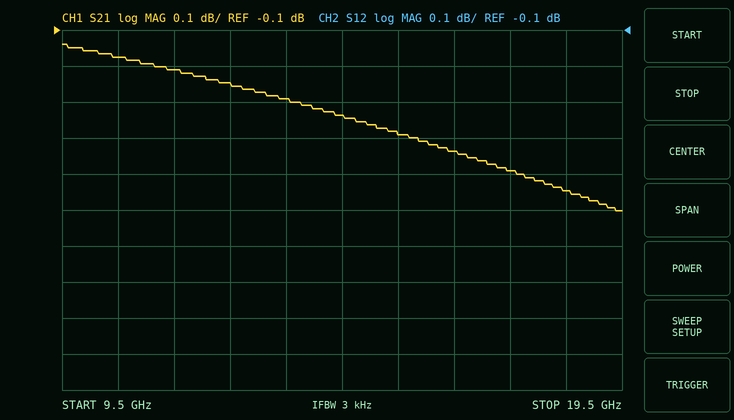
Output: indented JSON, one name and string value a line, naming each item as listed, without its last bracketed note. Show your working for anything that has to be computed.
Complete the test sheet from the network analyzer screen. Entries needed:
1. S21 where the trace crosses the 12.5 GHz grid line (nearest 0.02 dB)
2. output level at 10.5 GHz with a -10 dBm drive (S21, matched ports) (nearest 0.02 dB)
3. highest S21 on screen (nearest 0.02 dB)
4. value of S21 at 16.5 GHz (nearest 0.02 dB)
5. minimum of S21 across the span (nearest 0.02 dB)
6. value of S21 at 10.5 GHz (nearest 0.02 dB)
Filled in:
{
  "S21 where the trace crosses the 12.5 GHz grid line": "-0.24 dB",
  "output level at 10.5 GHz with a -10 dBm drive (S21, matched ports)": "-10 dBm + (-0.18 dB) = -10.18 dBm",
  "highest S21 on screen": "-0.14 dB",
  "value of S21 at 16.5 GHz": "-0.44 dB",
  "minimum of S21 across the span": "-0.60 dB",
  "value of S21 at 10.5 GHz": "-0.18 dB"
}
